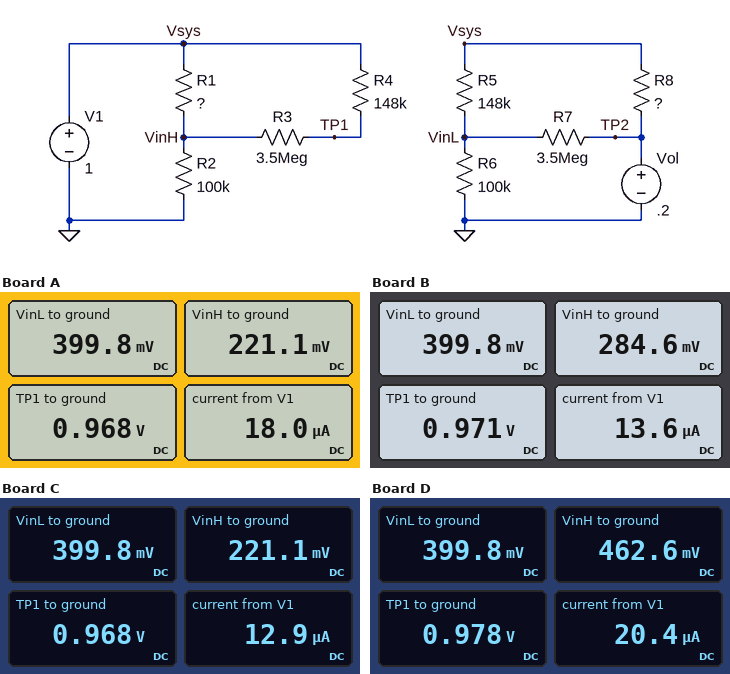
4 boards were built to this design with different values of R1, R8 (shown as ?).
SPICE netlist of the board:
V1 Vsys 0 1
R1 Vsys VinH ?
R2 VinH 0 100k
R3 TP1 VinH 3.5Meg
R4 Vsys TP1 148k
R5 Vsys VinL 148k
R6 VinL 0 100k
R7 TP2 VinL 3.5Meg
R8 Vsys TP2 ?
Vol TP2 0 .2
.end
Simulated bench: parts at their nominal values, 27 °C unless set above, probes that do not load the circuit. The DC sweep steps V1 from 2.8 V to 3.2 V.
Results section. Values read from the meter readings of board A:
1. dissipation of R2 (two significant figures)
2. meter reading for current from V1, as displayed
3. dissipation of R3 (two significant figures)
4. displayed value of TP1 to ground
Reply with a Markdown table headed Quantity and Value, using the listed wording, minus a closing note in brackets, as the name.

| Quantity | Value |
|---|---|
| dissipation of R2 | 490 nW |
| meter reading for current from V1, as displayed | 18.0 µA |
| dissipation of R3 | 160 nW |
| displayed value of TP1 to ground | 0.968 V |
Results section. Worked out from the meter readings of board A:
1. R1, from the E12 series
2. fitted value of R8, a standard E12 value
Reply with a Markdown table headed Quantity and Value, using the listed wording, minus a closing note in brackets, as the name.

| Quantity | Value |
|---|---|
| R1, from the E12 series | 390 kΩ |
| fitted value of R8, a standard E12 value | 68 kΩ |
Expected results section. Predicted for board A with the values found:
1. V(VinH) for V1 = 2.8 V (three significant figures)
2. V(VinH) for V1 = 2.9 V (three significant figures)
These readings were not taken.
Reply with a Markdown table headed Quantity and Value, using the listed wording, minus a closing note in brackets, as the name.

| Quantity | Value |
|---|---|
| V(VinH) for V1 = 2.8 V | 619 mV |
| V(VinH) for V1 = 2.9 V | 641 mV |
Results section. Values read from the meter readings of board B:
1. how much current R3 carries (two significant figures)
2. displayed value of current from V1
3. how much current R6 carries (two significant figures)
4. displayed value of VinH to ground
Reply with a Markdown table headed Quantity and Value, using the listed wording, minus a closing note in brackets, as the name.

| Quantity | Value |
|---|---|
| how much current R3 carries | 200 nA |
| displayed value of current from V1 | 13.6 µA |
| how much current R6 carries | 4.0 µA |
| displayed value of VinH to ground | 284.6 mV |
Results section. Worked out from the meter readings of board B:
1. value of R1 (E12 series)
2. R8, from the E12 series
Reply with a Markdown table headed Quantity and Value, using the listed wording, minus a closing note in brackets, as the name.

| Quantity | Value |
|---|---|
| value of R1 | 270 kΩ |
| R8, from the E12 series | 120 kΩ |
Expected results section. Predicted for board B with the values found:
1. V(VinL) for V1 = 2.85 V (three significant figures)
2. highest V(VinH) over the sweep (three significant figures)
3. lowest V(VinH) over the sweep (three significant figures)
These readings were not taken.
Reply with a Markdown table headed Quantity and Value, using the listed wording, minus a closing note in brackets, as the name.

| Quantity | Value |
|---|---|
| V(VinL) for V1 = 2.85 V | 1.13 V |
| highest V(VinH) over the sweep | 911 mV |
| lowest V(VinH) over the sweep | 797 mV |
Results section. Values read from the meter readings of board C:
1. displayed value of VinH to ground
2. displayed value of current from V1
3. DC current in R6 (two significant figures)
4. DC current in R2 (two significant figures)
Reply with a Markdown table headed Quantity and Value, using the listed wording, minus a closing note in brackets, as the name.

| Quantity | Value |
|---|---|
| displayed value of VinH to ground | 221.1 mV |
| displayed value of current from V1 | 12.9 µA |
| DC current in R6 | 4.0 µA |
| DC current in R2 | 2.2 µA |
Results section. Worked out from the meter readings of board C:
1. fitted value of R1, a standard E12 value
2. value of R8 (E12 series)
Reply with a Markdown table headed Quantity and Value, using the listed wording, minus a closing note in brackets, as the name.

| Quantity | Value |
|---|---|
| fitted value of R1, a standard E12 value | 390 kΩ |
| value of R8 | 120 kΩ |
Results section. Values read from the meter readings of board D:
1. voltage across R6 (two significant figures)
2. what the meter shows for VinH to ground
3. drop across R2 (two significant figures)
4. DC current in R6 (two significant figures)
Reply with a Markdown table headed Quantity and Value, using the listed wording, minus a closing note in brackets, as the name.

| Quantity | Value |
|---|---|
| voltage across R6 | 400 mV |
| what the meter shows for VinH to ground | 462.6 mV |
| drop across R2 | 460 mV |
| DC current in R6 | 4.0 µA |
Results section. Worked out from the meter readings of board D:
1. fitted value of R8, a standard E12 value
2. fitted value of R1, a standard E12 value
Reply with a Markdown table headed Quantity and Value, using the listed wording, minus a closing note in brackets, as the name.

| Quantity | Value |
|---|---|
| fitted value of R8, a standard E12 value | 68 kΩ |
| fitted value of R1, a standard E12 value | 120 kΩ |
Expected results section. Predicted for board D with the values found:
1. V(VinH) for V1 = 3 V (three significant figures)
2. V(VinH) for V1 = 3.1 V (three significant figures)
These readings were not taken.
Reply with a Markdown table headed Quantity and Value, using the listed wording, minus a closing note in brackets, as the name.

| Quantity | Value |
|---|---|
| V(VinH) for V1 = 3 V | 1.39 V |
| V(VinH) for V1 = 3.1 V | 1.43 V |
